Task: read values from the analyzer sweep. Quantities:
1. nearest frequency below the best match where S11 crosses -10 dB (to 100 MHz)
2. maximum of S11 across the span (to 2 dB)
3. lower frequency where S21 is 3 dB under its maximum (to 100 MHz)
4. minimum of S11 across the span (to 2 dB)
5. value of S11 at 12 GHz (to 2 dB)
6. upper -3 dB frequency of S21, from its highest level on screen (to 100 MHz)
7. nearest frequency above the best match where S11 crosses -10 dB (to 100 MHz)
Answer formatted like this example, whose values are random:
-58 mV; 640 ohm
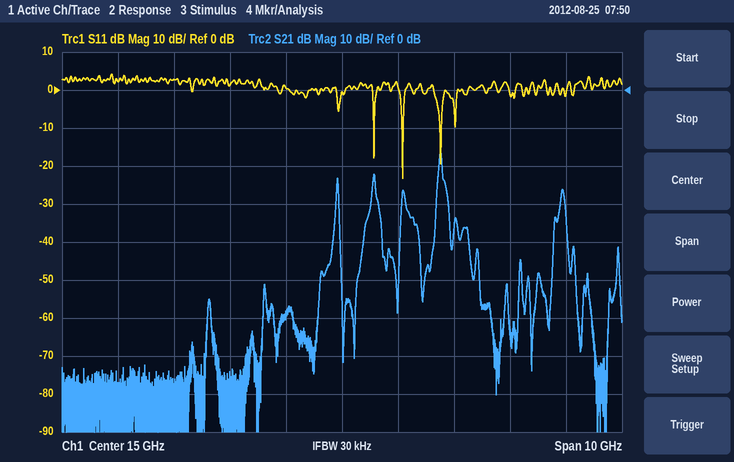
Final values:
16.1 GHz; 4 dB; 16.7 GHz; -24 dB; 2 dB; 16.8 GHz; 16.1 GHz
